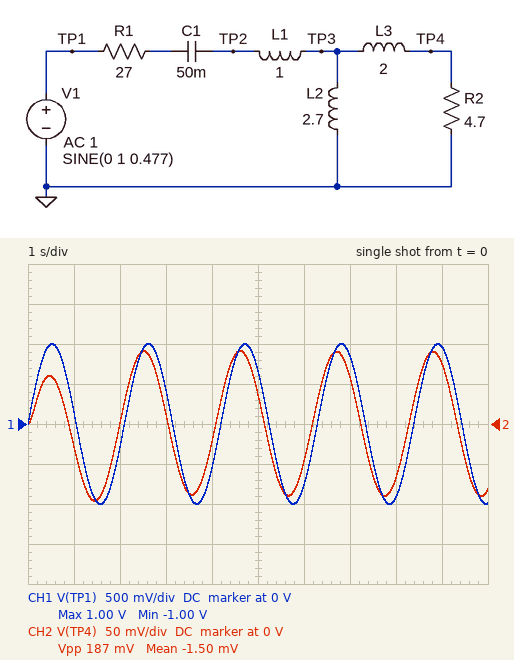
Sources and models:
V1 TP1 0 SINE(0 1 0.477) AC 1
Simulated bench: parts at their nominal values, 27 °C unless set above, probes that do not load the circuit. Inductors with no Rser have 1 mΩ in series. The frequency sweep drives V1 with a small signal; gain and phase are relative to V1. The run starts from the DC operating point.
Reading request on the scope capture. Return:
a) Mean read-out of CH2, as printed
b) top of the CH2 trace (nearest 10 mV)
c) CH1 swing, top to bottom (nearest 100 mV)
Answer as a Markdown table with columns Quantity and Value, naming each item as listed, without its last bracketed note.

| Quantity | Value |
|---|---|
| Mean read-out of CH2, as printed | -1.50 mV |
| top of the CH2 trace | 90 mV |
| CH1 swing, top to bottom | 2.0 V |
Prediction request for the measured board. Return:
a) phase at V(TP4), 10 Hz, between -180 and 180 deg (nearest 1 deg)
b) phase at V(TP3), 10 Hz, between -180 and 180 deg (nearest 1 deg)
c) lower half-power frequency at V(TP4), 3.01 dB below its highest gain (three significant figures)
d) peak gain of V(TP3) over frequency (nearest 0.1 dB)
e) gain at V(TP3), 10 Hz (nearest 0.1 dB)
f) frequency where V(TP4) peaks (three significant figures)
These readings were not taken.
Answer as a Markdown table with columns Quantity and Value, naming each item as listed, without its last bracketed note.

| Quantity | Value |
|---|---|
| phase at V(TP4), 10 Hz, between -180 and 180 deg | -77 deg |
| phase at V(TP3), 10 Hz, between -180 and 180 deg | 11 deg |
| lower half-power frequency at V(TP4), 3.01 dB below its highest gain | 180 mHz |
| peak gain of V(TP3) over frequency | -5.4 dB |
| gain at V(TP3), 10 Hz | -5.6 dB |
| frequency where V(TP4) peaks | 616 mHz |
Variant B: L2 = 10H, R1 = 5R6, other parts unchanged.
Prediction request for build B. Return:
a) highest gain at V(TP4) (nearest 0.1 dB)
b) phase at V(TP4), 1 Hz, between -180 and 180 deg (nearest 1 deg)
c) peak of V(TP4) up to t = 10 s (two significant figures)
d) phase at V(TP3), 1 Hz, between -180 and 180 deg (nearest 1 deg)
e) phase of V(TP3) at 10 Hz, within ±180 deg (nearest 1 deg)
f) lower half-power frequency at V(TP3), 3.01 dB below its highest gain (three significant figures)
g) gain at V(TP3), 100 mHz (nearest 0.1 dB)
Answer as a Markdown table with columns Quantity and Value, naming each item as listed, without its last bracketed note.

| Quantity | Value |
|---|---|
| highest gain at V(TP4) | -7.1 dB |
| phase at V(TP4), 1 Hz, between -180 and 180 deg | -54 deg |
| peak of V(TP4) up to t = 10 s | 440 mV |
| phase at V(TP3), 1 Hz, between -180 and 180 deg | 16 deg |
| phase of V(TP3) at 10 Hz, within ±180 deg | 1 deg |
| lower half-power frequency at V(TP3), 3.01 dB below its highest gain | 311 mHz |
| gain at V(TP3), 100 mHz | -18.7 dB |
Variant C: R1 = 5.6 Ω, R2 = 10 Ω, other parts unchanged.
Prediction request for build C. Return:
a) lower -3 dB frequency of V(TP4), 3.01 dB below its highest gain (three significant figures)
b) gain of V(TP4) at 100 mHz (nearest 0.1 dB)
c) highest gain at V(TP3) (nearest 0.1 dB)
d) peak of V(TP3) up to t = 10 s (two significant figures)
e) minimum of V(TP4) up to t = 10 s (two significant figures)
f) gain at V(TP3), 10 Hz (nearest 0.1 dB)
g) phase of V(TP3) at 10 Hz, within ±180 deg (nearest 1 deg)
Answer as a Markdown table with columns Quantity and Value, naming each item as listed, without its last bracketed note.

| Quantity | Value |
|---|---|
| lower -3 dB frequency of V(TP4), 3.01 dB below its highest gain | 289 mHz |
| gain of V(TP4) at 100 mHz | -25.4 dB |
| highest gain at V(TP3) | -3.2 dB |
| peak of V(TP3) up to t = 10 s | 700 mV |
| minimum of V(TP4) up to t = 10 s | -600 mV |
| gain at V(TP3), 10 Hz | -5.4 dB |
| phase of V(TP3) at 10 Hz, within ±180 deg | 1 deg |
